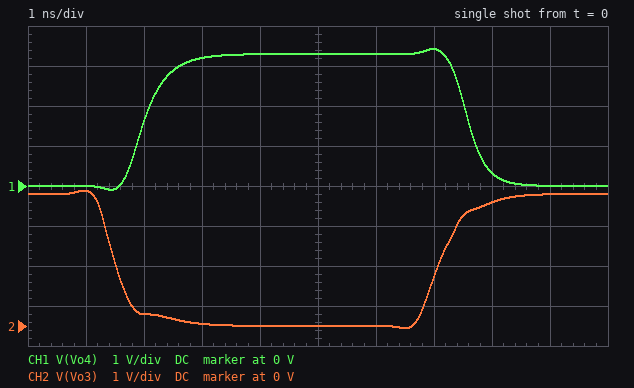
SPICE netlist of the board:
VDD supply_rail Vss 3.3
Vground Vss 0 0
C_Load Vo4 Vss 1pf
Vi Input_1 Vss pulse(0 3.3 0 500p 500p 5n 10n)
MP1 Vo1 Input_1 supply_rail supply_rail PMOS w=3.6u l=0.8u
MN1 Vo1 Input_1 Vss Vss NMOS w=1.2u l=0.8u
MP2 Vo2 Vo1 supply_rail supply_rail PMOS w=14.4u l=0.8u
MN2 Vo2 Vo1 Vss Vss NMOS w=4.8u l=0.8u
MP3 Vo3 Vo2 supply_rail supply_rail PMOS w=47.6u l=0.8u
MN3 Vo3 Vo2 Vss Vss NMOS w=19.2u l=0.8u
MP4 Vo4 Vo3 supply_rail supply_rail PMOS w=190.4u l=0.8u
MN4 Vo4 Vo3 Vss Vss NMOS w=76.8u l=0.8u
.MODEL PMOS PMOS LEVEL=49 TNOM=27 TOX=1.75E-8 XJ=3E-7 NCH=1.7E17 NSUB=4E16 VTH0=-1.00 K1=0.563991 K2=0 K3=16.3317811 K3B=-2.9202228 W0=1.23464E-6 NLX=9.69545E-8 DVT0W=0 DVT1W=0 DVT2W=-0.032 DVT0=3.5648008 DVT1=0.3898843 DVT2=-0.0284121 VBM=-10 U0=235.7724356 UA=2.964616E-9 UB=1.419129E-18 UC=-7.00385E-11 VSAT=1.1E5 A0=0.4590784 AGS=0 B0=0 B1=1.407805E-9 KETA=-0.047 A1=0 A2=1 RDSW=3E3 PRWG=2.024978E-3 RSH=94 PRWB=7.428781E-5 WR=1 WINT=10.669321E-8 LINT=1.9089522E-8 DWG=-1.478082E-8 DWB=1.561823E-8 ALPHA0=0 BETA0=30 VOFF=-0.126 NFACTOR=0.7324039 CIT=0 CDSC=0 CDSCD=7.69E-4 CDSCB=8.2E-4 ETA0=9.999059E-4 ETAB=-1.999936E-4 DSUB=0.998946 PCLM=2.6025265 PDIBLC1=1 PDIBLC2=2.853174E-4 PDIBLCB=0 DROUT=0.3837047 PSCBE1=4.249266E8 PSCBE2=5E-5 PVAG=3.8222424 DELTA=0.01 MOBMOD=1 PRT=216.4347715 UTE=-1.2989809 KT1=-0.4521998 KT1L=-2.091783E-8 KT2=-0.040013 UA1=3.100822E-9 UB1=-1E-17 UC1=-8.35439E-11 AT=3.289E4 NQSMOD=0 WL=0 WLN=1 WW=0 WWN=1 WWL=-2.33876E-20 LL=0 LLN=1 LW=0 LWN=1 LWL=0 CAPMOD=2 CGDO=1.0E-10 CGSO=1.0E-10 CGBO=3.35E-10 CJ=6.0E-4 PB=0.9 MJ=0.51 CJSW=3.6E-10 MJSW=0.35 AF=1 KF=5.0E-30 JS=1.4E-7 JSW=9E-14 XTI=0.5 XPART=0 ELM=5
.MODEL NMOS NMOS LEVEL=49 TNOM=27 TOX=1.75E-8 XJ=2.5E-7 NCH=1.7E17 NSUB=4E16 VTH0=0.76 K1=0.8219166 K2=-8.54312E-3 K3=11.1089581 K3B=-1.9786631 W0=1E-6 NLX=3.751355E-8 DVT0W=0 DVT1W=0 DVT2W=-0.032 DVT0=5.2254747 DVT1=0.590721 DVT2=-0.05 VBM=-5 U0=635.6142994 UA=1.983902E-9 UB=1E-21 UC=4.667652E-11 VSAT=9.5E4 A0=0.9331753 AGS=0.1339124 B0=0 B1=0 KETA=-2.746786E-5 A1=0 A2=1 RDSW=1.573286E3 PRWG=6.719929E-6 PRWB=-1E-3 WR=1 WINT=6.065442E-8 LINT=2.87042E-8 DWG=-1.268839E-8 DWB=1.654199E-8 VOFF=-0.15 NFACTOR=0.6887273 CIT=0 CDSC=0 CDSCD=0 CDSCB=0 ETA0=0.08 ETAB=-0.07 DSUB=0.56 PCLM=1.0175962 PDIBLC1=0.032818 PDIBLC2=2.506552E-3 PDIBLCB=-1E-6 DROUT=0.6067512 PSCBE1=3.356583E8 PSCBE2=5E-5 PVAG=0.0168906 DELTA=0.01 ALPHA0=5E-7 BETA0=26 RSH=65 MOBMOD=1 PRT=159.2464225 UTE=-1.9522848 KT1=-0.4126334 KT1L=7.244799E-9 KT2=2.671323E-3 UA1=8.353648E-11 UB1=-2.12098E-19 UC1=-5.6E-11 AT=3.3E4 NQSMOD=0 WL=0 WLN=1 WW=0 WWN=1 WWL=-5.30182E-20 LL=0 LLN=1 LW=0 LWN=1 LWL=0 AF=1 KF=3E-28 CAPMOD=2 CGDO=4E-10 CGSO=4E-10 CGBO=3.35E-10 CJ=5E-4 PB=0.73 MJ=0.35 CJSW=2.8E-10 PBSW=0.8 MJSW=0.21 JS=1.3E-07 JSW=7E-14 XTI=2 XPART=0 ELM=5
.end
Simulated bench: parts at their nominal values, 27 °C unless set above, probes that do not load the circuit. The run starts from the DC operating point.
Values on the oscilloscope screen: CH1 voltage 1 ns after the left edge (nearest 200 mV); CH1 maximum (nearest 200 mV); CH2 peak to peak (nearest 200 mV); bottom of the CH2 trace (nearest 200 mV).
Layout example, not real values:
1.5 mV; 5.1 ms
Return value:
0 V; 3.4 V; 3.4 V; 0 V
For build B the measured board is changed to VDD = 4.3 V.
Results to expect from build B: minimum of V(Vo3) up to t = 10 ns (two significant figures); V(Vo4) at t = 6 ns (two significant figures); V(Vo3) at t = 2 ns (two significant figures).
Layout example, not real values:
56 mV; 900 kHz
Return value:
-61 mV; 4.3 V; 430 mV
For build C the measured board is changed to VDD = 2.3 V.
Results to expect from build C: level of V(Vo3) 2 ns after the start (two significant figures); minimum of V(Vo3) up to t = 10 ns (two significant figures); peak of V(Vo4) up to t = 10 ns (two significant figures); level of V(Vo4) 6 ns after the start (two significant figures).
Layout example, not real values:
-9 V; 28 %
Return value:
650 mV; -48 mV; 2.4 V; 2.3 V
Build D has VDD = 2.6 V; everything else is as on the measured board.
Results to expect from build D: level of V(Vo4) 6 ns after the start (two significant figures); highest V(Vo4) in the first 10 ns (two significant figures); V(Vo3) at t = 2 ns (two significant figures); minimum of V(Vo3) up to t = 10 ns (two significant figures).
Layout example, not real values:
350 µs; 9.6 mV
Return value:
2.6 V; 2.7 V; 380 mV; -50 mV
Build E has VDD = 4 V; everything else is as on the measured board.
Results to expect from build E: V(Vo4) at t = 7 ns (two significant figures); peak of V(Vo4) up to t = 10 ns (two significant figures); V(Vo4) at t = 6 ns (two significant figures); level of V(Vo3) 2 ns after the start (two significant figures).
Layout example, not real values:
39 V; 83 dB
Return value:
3.7 V; 4.1 V; 4.0 V; 390 mV
